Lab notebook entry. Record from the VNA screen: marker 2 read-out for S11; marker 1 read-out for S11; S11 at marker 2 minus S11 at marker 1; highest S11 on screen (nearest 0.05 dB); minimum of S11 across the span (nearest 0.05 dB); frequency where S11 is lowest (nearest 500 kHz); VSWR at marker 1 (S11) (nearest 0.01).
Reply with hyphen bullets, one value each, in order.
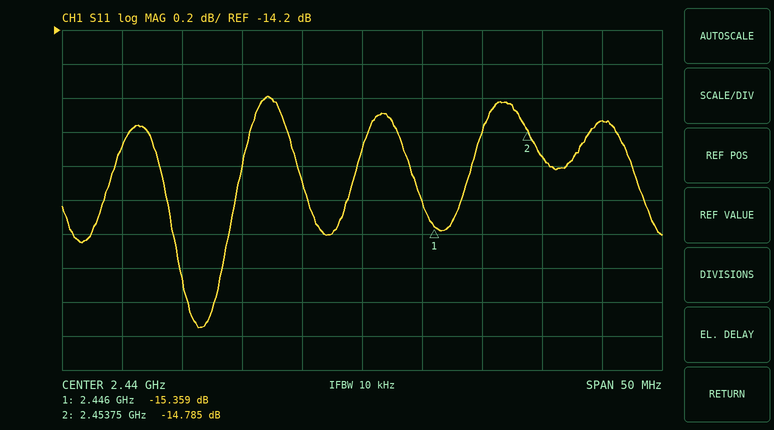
- -14.785 dB
- -15.359 dB
- 0.574 dB
- -14.60 dB
- -15.95 dB
- 2.4265 GHz
- 1.41
